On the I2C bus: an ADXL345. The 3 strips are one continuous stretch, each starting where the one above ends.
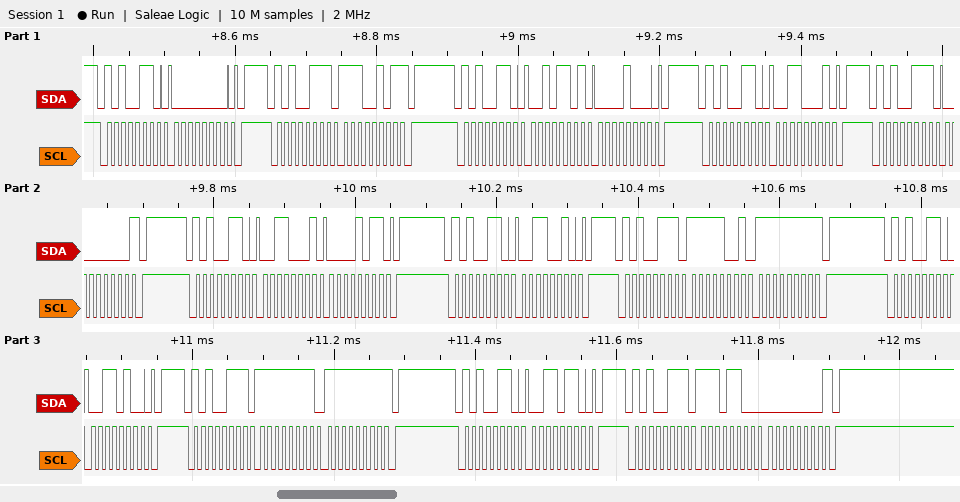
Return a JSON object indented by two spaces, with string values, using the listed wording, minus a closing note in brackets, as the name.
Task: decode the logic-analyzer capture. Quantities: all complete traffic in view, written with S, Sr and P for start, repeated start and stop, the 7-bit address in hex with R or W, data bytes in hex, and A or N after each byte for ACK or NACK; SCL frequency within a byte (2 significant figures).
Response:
{
  "all complete traffic in view, written with S, Sr and P for start, repeated start and stop, the 7-bit address in hex with R or W, data bytes in hex, and A or N after each byte for ACK or NACK": "S 53W A 00 A P S 53R A E5 N P S 53W A 2D A 08 A P S 53W A 31 A P S 53R A 00 N P S 53W A 31 A 0B A P S 53W A 32 A P S 53R A F9 A FF N P S 53W A 34 A P S 53R A FF A FF N P S 53W A 36 A P S 53R A EC A 00 N P",
  "SCL frequency within a byte": "100 kHz"
}
